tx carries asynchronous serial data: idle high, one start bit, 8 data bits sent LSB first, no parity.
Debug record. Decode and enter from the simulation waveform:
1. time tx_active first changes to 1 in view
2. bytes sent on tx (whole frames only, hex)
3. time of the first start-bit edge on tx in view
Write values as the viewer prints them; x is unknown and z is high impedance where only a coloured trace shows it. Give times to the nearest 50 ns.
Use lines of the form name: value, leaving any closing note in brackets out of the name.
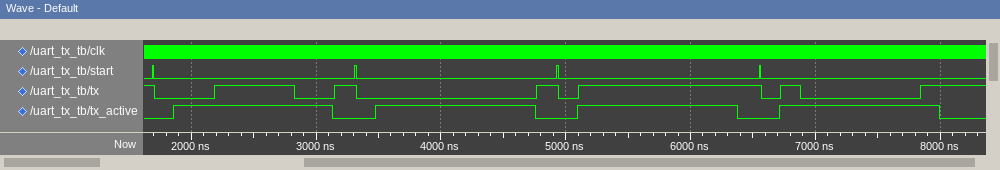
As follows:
time tx_active first changes to 1 in view: 1850 ns
bytes sent on tx: 3C, 00, FF, 81
time of the first start-bit edge on tx in view: 1700 ns
